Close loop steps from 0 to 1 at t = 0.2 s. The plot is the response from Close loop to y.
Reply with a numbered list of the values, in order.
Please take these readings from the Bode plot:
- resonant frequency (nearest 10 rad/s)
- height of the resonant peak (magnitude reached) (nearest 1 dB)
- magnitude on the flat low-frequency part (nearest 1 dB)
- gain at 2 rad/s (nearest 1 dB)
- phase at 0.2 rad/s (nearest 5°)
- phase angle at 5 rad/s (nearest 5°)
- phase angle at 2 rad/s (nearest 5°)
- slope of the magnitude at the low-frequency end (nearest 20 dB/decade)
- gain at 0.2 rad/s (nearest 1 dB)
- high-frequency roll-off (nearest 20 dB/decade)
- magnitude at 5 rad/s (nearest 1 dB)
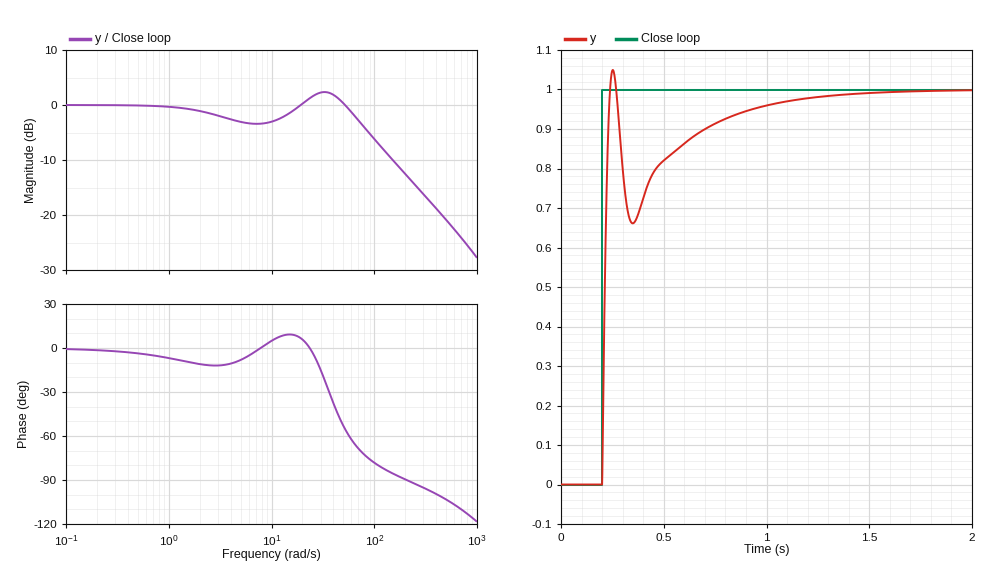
1. 30 rad/s
2. 2 dB
3. 0 dB
4. -1 dB
5. 0°
6. -10°
7. -10°
8. 0 dB/decade
9. 0 dB
10. -20 dB/decade
11. -3 dB
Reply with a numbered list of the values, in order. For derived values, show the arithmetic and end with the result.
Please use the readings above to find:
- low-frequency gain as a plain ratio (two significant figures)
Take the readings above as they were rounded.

1. 10^(0 / 20) = 1.0
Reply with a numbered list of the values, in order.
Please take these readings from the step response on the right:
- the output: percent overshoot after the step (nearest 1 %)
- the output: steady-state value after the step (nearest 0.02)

1. 5 %
2. 1.00
